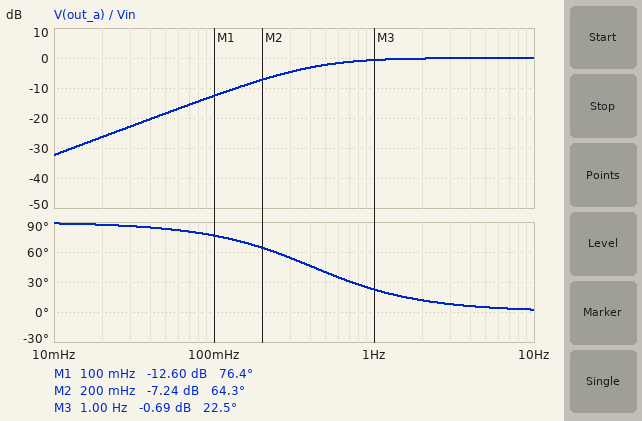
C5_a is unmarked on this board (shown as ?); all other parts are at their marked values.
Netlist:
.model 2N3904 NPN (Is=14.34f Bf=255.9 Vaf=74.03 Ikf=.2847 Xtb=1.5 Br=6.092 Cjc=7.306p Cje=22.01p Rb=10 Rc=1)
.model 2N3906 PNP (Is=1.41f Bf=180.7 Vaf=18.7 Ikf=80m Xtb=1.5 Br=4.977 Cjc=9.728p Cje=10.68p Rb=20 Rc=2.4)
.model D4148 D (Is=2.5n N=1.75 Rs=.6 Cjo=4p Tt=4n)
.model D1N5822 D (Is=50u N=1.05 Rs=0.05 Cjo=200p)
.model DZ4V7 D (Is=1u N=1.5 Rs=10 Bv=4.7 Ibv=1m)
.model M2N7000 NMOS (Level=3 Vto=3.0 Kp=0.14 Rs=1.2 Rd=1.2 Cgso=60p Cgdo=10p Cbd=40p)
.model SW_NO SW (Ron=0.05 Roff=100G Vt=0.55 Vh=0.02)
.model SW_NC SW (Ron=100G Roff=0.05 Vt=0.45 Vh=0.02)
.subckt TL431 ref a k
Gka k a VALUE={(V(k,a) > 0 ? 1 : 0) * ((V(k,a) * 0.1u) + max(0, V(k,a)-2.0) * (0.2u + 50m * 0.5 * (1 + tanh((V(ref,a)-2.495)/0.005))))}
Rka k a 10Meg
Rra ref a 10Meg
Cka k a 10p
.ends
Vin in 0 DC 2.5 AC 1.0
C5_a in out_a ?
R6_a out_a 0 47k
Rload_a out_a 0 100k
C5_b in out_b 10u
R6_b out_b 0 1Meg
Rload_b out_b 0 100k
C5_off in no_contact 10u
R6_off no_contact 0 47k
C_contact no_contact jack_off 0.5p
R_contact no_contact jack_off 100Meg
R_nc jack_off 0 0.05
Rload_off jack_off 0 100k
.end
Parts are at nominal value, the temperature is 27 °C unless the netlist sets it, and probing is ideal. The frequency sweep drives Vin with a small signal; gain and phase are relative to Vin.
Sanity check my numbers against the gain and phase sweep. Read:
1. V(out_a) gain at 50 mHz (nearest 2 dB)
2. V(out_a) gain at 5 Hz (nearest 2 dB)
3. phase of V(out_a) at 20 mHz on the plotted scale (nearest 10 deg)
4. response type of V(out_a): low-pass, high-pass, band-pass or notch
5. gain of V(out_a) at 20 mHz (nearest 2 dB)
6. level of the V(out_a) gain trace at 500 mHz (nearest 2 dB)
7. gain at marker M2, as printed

-18 dB
0 dB
90 deg
high-pass
-26 dB
-2 dB
-7.24 dB
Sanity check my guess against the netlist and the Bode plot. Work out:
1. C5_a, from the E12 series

12 µF
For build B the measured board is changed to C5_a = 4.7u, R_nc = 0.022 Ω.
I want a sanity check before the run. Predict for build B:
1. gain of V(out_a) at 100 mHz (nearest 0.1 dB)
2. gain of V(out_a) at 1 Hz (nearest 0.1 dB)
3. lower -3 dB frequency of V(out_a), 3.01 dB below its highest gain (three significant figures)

-20.5 dB
-3.3 dB
1.06 Hz
